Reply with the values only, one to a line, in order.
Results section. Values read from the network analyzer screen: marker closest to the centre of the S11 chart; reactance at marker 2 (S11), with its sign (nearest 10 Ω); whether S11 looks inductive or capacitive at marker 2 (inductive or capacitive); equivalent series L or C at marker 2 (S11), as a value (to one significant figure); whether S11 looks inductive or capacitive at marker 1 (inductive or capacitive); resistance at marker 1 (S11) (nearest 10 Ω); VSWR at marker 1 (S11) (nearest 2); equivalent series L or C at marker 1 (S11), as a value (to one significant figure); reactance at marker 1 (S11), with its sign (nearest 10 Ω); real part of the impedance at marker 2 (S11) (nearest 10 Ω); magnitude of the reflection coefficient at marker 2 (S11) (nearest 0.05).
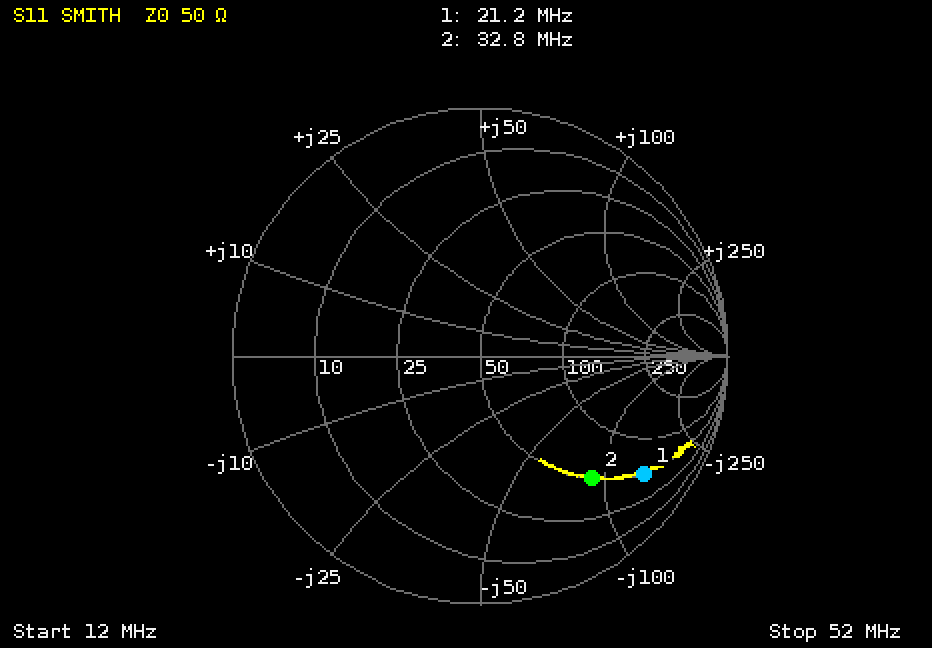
marker 2
-90 Ω
capacitive
50 pF
capacitive
50 Ω
10
50 pF
-140 Ω
50 Ω
0.65
